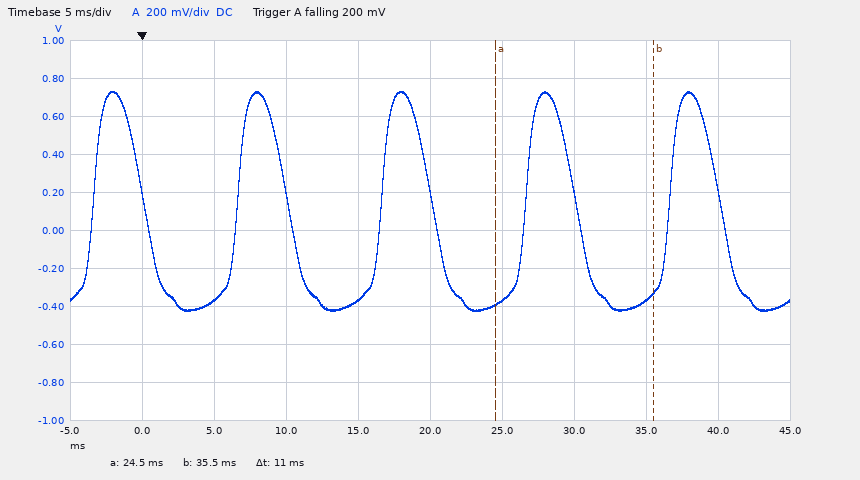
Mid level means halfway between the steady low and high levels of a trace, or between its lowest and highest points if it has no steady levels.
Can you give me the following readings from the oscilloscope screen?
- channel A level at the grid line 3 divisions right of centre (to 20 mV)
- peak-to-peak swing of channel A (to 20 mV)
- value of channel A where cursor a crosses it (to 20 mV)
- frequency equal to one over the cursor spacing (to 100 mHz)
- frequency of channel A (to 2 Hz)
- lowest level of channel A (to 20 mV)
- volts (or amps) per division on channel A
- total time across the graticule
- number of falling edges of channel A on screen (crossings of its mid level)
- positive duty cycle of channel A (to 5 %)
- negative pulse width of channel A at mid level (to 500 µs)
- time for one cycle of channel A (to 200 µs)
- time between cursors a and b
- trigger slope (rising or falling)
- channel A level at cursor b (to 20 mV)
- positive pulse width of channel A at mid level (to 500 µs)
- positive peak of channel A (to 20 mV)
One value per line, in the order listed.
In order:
-360 mV
1.16 V
-380 mV
90.9 Hz
100 Hz
-420 mV
200 mV
50 ms
5
35 %
6.5 ms
10.0 ms
11 ms
falling
-320 mV
3.5 ms
740 mV
